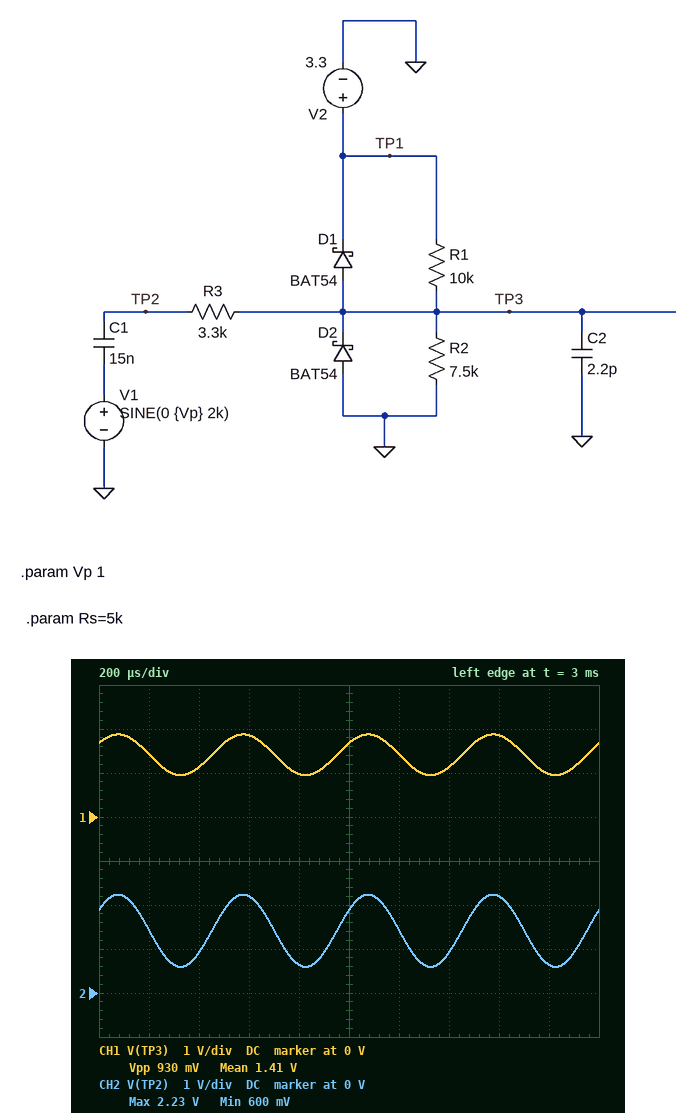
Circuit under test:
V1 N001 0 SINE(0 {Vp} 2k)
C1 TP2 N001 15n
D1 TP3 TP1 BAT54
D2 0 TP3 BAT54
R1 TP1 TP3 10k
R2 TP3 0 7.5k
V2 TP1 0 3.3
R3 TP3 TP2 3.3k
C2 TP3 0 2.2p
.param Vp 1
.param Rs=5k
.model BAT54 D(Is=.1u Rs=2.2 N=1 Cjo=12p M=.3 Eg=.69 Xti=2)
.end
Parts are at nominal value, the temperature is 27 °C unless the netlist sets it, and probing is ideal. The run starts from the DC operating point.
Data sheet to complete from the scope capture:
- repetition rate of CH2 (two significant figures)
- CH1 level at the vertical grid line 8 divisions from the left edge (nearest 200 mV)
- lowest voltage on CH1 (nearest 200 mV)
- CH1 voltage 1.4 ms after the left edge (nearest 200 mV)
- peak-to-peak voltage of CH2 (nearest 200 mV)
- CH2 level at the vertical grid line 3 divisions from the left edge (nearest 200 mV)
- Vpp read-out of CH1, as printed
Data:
2.0 kHz
1.8 V
1.0 V
1.2 V
1.6 V
2.2 V
930 mV
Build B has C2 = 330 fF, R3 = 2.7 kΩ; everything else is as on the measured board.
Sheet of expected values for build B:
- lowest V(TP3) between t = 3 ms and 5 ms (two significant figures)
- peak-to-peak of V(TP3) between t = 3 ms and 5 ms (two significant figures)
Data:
930 mV
980 mV
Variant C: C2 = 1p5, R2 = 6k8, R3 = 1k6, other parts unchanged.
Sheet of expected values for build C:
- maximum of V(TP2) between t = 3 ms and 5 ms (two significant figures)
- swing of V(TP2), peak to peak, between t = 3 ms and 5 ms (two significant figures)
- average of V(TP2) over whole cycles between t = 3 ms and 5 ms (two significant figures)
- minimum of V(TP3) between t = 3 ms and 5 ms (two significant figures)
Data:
2.1 V
1.5 V
1.3 V
810 mV
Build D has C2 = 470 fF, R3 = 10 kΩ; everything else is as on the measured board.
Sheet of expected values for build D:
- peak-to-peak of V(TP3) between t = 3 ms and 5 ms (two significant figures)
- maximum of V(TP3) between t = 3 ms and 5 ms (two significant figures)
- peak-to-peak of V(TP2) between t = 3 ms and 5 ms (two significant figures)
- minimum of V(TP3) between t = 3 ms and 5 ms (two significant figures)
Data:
560 mV
1.7 V
1.9 V
1.1 V
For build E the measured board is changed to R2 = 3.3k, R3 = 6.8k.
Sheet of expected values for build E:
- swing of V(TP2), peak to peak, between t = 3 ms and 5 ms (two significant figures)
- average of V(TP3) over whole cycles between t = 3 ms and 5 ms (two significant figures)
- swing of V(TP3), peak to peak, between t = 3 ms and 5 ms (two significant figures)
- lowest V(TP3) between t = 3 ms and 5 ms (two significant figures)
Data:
1.7 V
820 mV
460 mV
590 mV
